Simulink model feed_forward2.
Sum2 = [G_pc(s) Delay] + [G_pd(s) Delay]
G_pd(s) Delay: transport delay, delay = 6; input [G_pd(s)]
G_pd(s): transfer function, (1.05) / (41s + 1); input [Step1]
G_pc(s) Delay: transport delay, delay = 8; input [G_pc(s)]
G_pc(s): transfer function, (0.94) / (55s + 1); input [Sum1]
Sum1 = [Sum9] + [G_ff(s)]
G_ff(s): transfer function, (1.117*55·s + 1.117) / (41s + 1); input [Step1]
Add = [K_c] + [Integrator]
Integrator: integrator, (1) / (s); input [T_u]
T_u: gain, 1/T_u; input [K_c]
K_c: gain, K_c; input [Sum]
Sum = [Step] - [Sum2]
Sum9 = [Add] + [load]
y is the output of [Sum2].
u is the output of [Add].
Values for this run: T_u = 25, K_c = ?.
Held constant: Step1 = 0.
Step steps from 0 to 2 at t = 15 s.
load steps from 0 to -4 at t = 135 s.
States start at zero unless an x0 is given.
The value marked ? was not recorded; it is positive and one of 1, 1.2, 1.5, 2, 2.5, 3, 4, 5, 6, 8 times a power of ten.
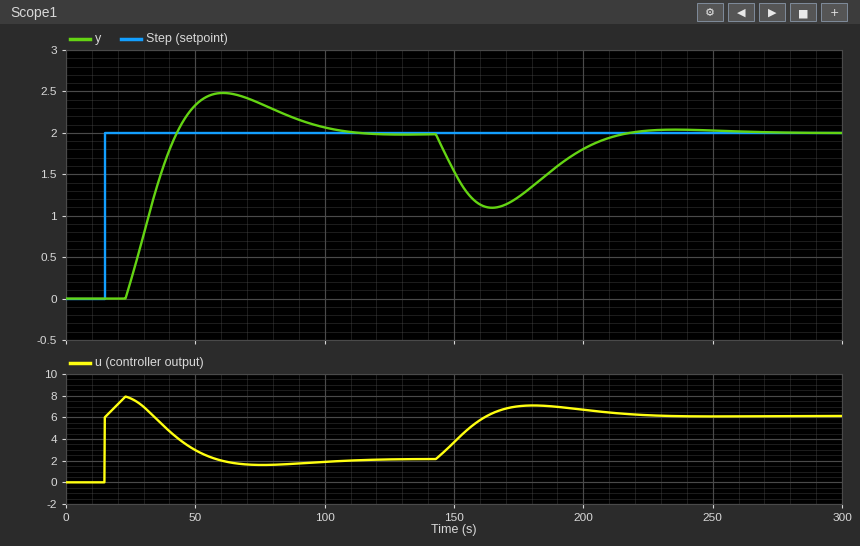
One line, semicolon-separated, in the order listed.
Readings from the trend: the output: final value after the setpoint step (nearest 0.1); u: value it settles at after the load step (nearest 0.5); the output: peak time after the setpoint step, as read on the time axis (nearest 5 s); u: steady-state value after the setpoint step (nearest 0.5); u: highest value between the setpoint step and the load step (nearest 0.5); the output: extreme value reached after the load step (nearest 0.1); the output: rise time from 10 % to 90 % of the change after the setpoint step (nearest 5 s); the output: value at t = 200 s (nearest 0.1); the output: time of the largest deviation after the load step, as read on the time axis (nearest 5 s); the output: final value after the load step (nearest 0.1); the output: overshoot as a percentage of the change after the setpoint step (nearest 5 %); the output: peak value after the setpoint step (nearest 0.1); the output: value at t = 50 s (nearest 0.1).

2.0; 6.0; 60 s; 2.0; 8.0; 1.1; 15 s; 1.8; 165 s; 2.0; 25 %; 2.5; 2.3
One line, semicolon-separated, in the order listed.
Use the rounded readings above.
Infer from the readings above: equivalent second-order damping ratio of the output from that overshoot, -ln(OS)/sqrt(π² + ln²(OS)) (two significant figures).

0.40
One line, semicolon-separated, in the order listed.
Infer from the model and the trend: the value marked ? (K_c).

3
